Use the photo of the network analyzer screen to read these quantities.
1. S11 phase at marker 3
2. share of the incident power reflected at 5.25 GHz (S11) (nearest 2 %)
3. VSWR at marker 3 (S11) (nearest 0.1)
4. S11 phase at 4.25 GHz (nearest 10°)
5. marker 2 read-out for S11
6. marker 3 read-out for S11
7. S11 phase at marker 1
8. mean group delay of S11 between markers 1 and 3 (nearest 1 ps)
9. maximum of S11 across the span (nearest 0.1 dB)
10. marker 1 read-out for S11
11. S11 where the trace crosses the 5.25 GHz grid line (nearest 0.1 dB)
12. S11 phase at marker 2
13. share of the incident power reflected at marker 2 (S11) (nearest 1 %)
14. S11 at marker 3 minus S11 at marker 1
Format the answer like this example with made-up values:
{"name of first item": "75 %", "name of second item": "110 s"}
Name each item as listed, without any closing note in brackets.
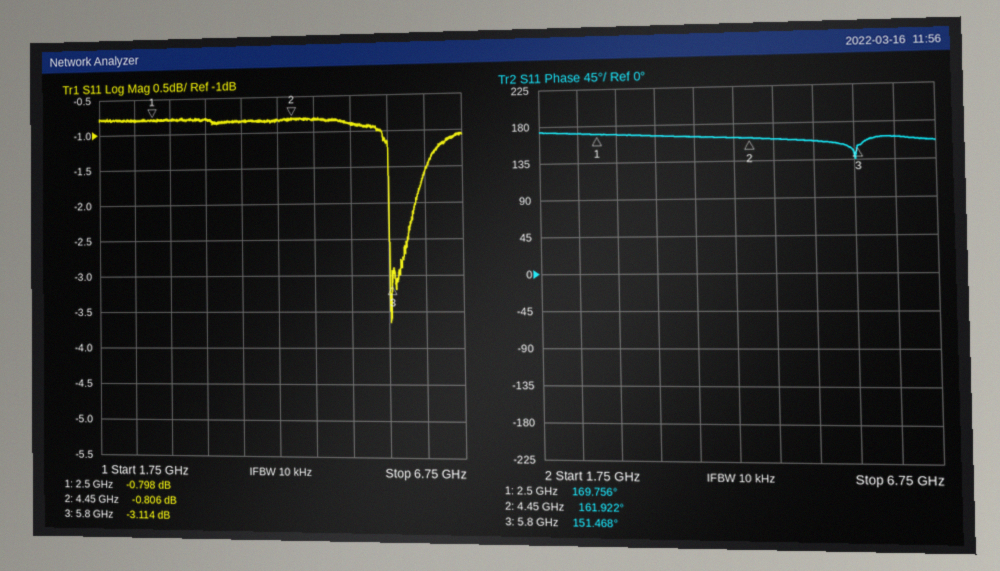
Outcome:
{"S11 phase at marker 3": "151.468°", "share of the incident power reflected at 5.25 GHz (S11)": "82 %", "VSWR at marker 3 (S11)": "5.6", "S11 phase at 4.25 GHz": "160°", "marker 2 read-out for S11": "-0.806 dB", "marker 3 read-out for S11": "-3.114 dB", "S11 phase at marker 1": "169.756°", "mean group delay of S11 between markers 1 and 3": "15 ps", "maximum of S11 across the span": "-0.8 dB", "marker 1 read-out for S11": "-0.798 dB", "S11 where the trace crosses the 5.25 GHz grid line": "-0.9 dB", "S11 phase at marker 2": "161.922°", "share of the incident power reflected at marker 2 (S11)": "83 %", "S11 at marker 3 minus S11 at marker 1": "-2.316 dB"}
